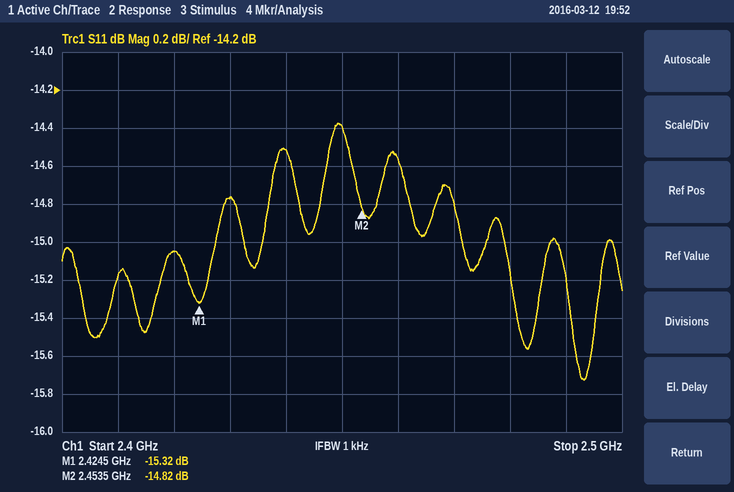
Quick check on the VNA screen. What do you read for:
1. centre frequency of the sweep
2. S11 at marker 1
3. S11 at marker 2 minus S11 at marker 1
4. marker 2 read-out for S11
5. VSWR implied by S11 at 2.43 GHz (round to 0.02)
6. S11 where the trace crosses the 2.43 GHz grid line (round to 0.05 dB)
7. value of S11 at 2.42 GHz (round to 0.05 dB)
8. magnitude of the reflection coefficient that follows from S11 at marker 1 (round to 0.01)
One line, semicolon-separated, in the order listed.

2.45 GHz; -15.32 dB; 0.50 dB; -14.82 dB; 1.44; -14.75 dB; -15.05 dB; 0.17
